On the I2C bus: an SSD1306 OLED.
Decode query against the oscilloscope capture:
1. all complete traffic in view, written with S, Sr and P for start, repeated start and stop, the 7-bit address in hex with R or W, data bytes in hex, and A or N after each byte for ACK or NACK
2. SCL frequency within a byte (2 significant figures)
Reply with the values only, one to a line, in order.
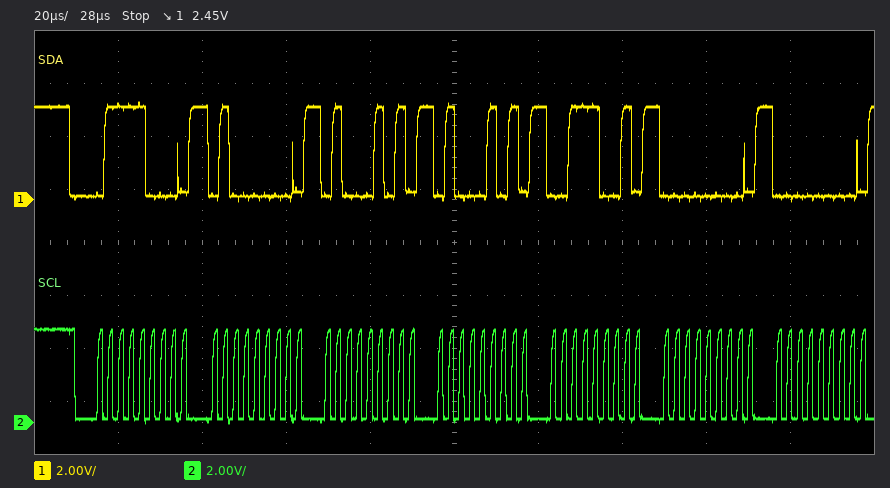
S 3CW A 40 A 45 A 45 A 39 A 00 A 00 A
400 kHz
